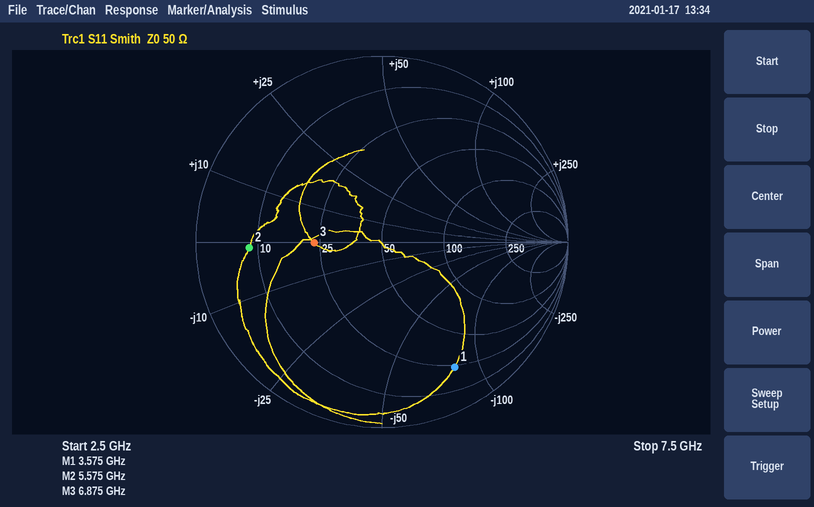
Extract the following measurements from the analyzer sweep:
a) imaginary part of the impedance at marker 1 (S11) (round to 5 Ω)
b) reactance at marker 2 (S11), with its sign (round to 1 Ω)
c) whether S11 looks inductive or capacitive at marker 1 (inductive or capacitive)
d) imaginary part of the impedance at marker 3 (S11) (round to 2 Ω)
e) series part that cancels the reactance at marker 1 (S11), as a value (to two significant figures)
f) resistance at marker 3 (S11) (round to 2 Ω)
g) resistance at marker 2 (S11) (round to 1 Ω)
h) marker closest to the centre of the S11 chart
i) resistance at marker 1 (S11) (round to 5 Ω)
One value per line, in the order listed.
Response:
-80 Ω
-1 Ω
capacitive
0 Ω
3.6 nH
24 Ω
8 Ω
marker 3
25 Ω
